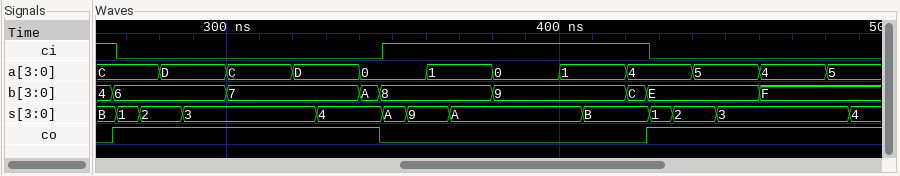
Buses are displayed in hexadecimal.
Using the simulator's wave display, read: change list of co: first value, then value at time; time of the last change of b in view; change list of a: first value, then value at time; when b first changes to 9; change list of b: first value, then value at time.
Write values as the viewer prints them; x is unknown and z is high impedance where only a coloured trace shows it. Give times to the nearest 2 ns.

0, 1 at 266 ns, 0 at 346 ns, 1 at 426 ns
460 ns
C, D at 280 ns, C at 300 ns, D at 320 ns, 0 at 340 ns, 1 at 360 ns, 0 at 380 ns, 1 at 400 ns, 4 at 420 ns, 5 at 440 ns, 4 at 460 ns, 5 at 480 ns
380 ns
4, 6 at 266 ns, 7 at 300 ns, A at 340 ns, 8 at 346 ns, 9 at 380 ns, C at 420 ns, E at 426 ns, F at 460 ns
